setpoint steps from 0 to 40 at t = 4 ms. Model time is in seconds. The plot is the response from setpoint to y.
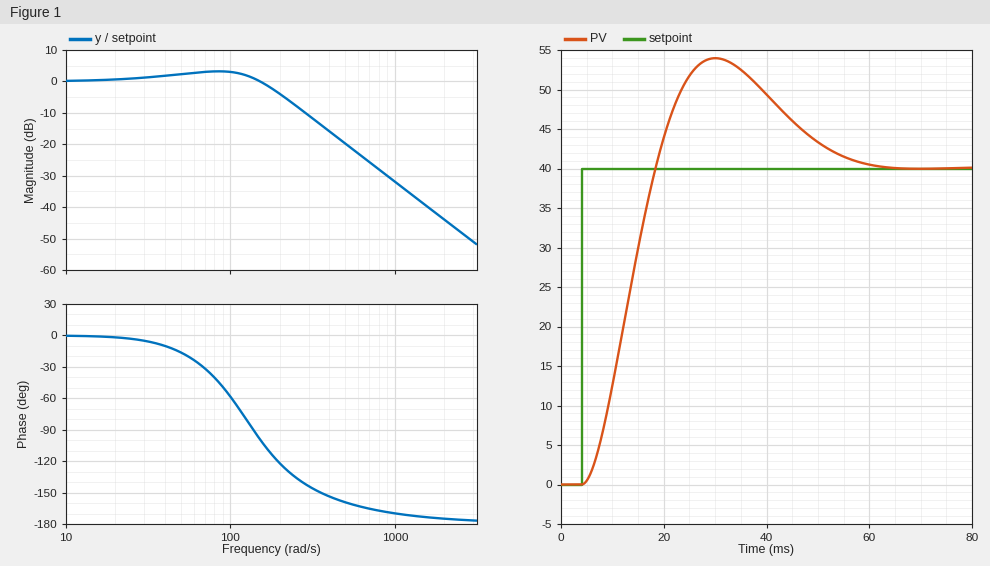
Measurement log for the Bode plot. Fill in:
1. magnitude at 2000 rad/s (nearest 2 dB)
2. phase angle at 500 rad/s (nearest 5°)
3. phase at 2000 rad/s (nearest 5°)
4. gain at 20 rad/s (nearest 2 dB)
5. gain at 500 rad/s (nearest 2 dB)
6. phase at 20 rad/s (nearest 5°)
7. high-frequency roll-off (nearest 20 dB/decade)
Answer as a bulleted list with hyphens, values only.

- -44 dB
- -160°
- -175°
- 0 dB
- -20 dB
- 0°
- -40 dB/decade
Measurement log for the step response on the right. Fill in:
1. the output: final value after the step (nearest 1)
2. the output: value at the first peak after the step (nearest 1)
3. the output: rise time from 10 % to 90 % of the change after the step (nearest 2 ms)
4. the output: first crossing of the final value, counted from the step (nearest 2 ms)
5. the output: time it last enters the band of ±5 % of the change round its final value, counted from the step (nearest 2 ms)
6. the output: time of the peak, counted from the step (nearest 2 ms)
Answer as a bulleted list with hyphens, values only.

- 40
- 54
- 10 ms
- 14 ms
- 50 ms
- 26 ms
